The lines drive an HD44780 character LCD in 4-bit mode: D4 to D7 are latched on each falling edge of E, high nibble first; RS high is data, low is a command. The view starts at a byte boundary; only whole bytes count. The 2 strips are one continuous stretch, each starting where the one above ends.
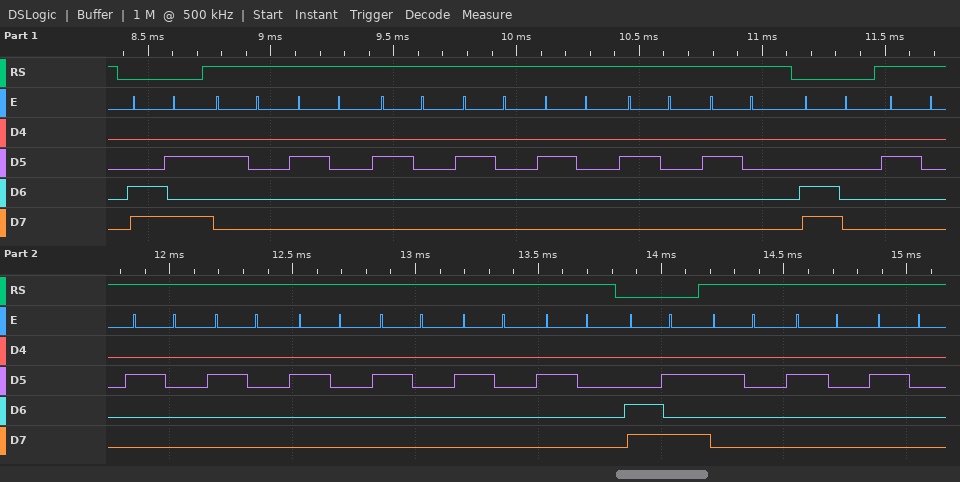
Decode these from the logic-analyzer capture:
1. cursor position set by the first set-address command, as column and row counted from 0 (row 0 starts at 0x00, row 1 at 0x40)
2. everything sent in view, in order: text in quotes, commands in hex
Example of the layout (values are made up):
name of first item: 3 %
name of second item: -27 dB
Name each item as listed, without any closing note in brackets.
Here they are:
cursor position set by the first set-address command, as column and row counted from 0: column 10, row 1
everything sent in view, in order: text in quotes, commands in hex: 0xCA "       " 0xC0 "       " 0xCA "   "
